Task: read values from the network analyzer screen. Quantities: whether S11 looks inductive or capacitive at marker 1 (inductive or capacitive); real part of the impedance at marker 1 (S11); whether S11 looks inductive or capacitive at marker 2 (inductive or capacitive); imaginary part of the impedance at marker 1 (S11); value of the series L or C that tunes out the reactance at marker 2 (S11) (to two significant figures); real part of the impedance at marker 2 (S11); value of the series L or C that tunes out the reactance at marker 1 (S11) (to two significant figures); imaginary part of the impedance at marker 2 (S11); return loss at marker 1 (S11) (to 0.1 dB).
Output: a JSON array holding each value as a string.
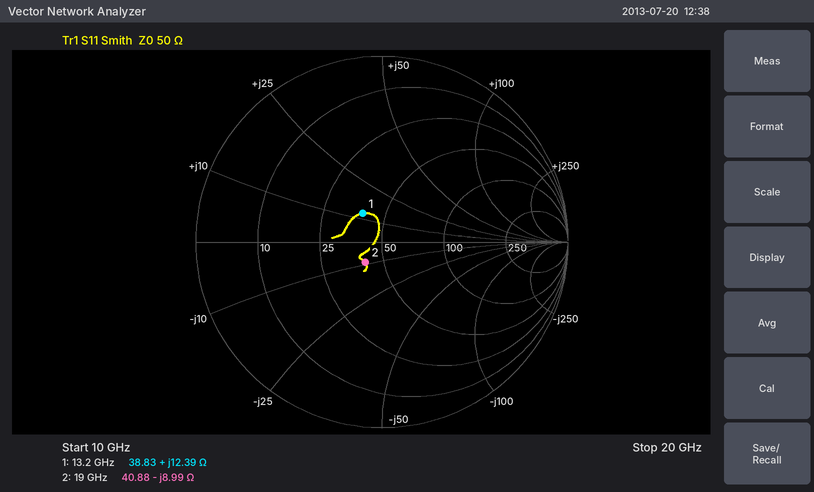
["inductive", "38.83 Ω", "capacitive", "+12.39 Ω", "75 pH", "40.88 Ω", "970 fF", "-8.99 Ω", "14.6 dB"]
